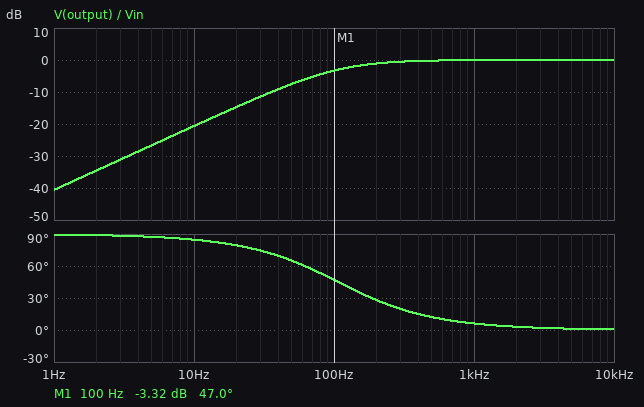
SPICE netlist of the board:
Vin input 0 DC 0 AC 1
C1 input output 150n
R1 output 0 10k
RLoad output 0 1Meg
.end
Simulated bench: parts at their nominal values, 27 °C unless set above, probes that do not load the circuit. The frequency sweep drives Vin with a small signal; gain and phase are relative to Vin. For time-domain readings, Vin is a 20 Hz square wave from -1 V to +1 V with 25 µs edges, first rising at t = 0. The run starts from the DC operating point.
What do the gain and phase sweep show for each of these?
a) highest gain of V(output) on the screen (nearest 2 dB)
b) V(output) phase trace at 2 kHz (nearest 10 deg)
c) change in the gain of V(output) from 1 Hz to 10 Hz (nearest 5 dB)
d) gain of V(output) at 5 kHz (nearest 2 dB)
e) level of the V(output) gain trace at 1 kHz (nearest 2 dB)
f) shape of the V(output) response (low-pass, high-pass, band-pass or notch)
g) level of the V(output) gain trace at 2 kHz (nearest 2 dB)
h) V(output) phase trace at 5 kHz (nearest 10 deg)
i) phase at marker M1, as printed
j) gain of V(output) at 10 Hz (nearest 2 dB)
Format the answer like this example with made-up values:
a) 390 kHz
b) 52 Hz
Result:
a) 0 dB
b) 0 deg
c) 20 dB
d) 0 dB
e) 0 dB
f) high-pass
g) 0 dB
h) 0 deg
i) 47.0 deg
j) -20 dB
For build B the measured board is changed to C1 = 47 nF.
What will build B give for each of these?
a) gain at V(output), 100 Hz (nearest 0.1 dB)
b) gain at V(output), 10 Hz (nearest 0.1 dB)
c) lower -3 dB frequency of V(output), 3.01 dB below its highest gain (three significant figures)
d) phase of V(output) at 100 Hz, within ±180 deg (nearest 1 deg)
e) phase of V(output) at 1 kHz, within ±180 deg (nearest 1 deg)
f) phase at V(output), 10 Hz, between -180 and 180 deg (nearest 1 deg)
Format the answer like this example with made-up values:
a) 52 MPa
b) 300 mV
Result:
a) -11.0 dB
b) -30.7 dB
c) 342 Hz
d) 74 deg
e) 19 deg
f) 88 deg
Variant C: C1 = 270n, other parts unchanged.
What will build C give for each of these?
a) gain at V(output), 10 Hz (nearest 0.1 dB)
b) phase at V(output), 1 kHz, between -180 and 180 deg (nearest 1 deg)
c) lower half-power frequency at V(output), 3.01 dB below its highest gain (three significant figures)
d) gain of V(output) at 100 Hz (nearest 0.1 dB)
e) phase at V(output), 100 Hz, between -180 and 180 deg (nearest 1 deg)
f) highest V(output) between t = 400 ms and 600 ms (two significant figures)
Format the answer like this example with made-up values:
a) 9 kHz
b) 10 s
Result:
a) -15.6 dB
b) 3 deg
c) 59.5 Hz
d) -1.3 dB
e) 31 deg
f) 2.0 V
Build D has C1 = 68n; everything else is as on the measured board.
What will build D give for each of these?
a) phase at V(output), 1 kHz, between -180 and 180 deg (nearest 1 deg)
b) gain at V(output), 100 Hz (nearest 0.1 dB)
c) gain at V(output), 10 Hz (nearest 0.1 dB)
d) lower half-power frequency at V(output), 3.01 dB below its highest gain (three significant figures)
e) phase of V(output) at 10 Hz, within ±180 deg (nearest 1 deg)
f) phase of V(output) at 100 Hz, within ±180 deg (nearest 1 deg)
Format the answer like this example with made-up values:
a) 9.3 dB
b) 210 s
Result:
a) 13 deg
b) -8.2 dB
c) -27.5 dB
d) 236 Hz
e) 88 deg
f) 67 deg
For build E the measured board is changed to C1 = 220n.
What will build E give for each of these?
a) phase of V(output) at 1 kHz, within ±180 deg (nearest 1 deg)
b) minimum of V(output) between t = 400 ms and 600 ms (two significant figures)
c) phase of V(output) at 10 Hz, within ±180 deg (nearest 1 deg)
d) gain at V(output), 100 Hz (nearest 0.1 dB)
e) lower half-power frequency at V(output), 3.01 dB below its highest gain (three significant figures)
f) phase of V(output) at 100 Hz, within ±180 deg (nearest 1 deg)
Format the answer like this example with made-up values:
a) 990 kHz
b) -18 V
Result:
a) 4 deg
b) -2.0 V
c) 82 deg
d) -1.9 dB
e) 73.1 Hz
f) 36 deg
